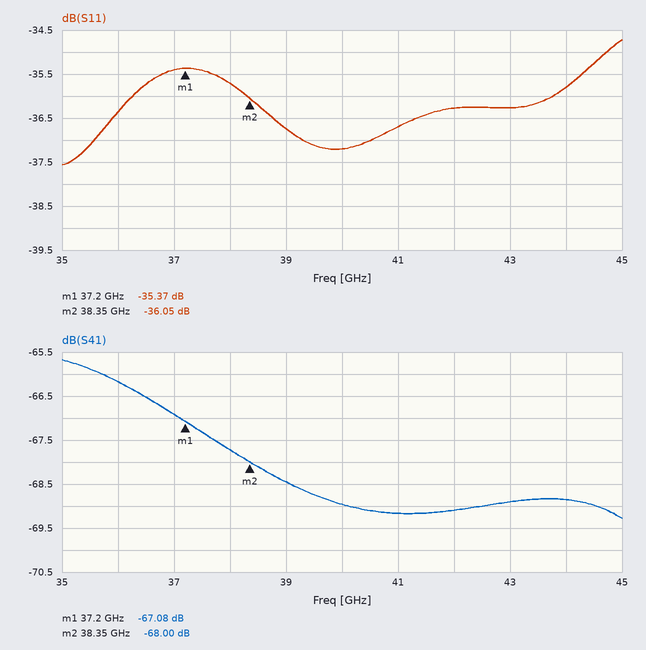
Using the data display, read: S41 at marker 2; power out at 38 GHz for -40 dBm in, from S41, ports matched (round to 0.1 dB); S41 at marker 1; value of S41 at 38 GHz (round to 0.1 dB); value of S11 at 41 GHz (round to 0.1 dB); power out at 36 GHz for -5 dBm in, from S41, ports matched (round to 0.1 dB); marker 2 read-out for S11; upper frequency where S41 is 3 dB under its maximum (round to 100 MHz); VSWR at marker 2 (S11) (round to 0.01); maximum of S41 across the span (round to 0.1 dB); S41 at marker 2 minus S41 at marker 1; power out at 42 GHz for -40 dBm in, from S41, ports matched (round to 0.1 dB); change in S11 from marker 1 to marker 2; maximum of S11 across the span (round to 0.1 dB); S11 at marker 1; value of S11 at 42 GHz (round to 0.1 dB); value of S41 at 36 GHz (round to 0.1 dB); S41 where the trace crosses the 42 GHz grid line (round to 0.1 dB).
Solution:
-68.00 dB
-107.7 dBm
-67.08 dB
-67.7 dB
-36.7 dB
-71.2 dBm
-36.05 dB
39.4 GHz
1.03
-65.7 dB
-0.92 dB
-109.1 dBm
-0.68 dB
-34.7 dB
-35.37 dB
-36.3 dB
-66.2 dB
-69.1 dB
